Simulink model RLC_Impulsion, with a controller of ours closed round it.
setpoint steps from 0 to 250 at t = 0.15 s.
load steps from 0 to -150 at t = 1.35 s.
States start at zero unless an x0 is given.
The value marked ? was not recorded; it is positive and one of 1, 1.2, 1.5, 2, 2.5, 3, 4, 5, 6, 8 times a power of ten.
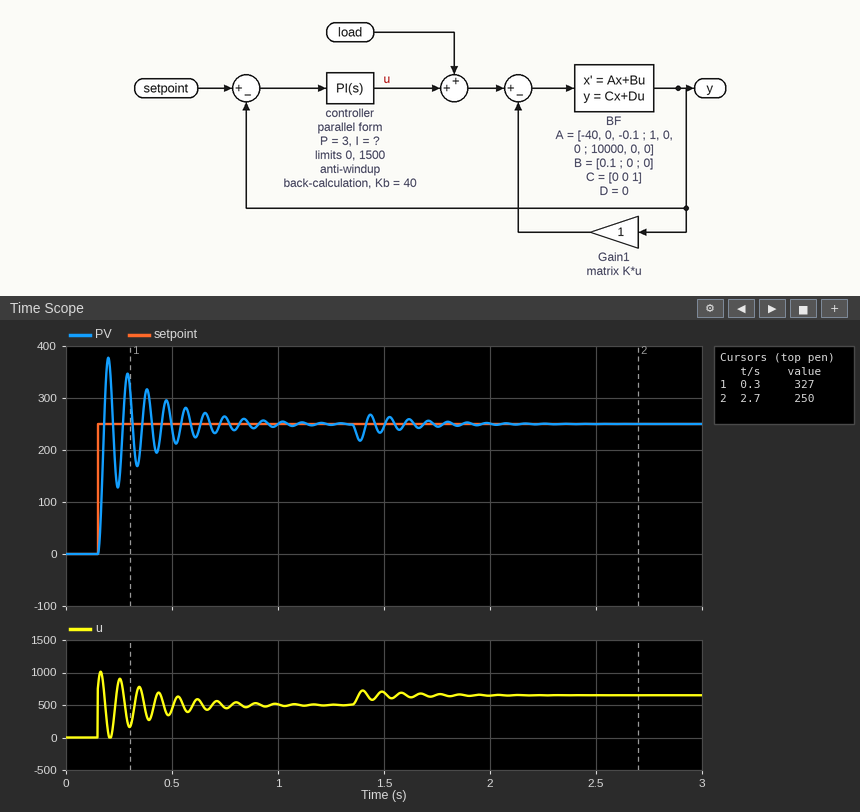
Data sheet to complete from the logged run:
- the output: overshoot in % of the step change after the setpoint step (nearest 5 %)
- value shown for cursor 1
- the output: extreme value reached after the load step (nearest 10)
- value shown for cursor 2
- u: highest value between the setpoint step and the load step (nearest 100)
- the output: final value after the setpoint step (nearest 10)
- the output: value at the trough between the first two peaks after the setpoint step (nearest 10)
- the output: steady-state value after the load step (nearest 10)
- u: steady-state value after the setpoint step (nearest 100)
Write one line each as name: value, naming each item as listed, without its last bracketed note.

the output: overshoot in % of the step change after the setpoint step: 50 %
value shown for cursor 1: 327
the output: extreme value reached after the load step: 220
value shown for cursor 2: 250
u: highest value between the setpoint step and the load step: 1000
the output: final value after the setpoint step: 250
the output: value at the trough between the first two peaks after the setpoint step: 130
the output: steady-state value after the load step: 250
u: steady-state value after the setpoint step: 500
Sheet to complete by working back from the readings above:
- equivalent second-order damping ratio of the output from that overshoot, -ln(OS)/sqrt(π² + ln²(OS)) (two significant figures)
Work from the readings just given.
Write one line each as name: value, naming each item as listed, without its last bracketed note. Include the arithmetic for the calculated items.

equivalent second-order damping ratio of the output from that overshoot, -ln(OS)/sqrt(π² + ln²(OS)): ln(0.5) = -0.693; 0.693 / sqrt(9.870 + 0.480) = 0.22
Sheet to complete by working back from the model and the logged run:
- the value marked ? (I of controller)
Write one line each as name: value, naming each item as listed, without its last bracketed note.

the value marked ?: 150
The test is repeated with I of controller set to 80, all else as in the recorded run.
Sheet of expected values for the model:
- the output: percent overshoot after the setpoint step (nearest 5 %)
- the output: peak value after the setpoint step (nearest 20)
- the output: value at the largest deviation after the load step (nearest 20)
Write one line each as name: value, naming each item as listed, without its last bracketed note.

the output: percent overshoot after the setpoint step: 25 %
the output: peak value after the setpoint step: 300
the output: value at the largest deviation after the load step: 220
